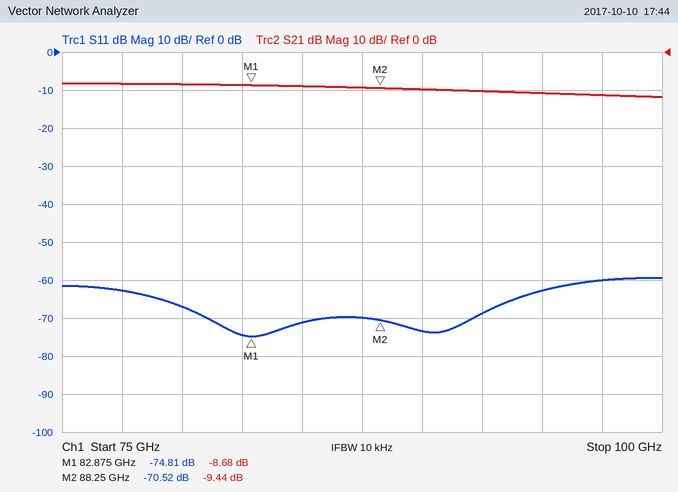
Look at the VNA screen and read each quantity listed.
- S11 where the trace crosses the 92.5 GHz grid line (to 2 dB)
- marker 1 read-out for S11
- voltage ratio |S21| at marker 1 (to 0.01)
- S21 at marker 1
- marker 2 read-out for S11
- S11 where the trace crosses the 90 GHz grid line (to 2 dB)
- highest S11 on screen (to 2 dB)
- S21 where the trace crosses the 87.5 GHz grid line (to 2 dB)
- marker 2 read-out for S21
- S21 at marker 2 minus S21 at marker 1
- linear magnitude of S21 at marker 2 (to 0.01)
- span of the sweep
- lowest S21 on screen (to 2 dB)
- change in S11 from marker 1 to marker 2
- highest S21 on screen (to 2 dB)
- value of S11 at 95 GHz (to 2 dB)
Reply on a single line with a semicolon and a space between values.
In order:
-68 dB; -74.81 dB; 0.37; -8.68 dB; -70.52 dB; -74 dB; -60 dB; -10 dB; -9.44 dB; -0.76 dB; 0.34; 25 GHz; -12 dB; 4.29 dB; -8 dB; -62 dB
